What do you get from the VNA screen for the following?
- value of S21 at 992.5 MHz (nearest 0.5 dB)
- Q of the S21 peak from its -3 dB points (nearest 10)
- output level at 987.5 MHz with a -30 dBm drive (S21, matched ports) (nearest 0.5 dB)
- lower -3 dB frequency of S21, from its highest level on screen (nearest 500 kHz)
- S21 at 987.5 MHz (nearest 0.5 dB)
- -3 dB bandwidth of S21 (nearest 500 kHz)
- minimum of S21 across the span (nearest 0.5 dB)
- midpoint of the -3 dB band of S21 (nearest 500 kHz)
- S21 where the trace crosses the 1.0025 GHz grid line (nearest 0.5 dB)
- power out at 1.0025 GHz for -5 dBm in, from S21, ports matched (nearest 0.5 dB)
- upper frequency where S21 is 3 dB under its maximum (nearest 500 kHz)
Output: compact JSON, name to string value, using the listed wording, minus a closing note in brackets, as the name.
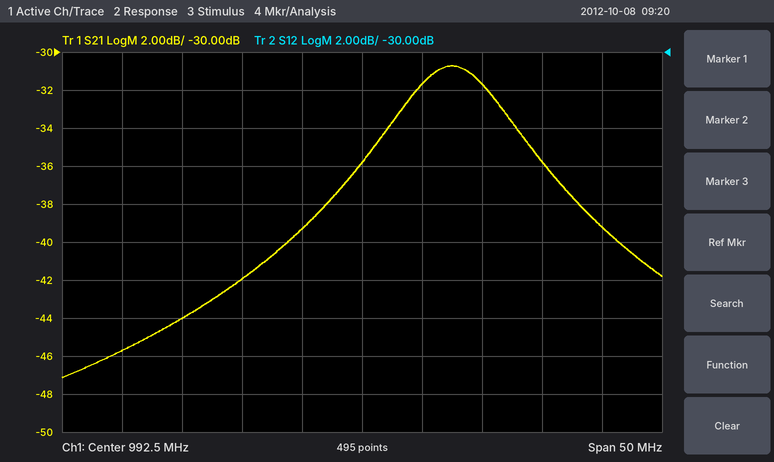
{"value of S21 at 992.5 MHz": "-36.0 dB", "Q of the S21 peak from its -3 dB points": "100", "output level at 987.5 MHz with a -30 dBm drive (S21, matched ports)": "-69.5 dBm", "lower -3 dB frequency of S21, from its highest level on screen": "995.0 MHz", "S21 at 987.5 MHz": "-39.5 dB", "-3 dB bandwidth of S21": "10.0 MHz", "minimum of S21 across the span": "-47.0 dB", "midpoint of the -3 dB band of S21": "1.0000 GHz", "S21 where the trace crosses the 1.0025 GHz grid line": "-31.5 dB", "power out at 1.0025 GHz for -5 dBm in, from S21, ports matched": "-36.5 dBm", "upper frequency where S21 is 3 dB under its maximum": "1.0050 GHz"}
